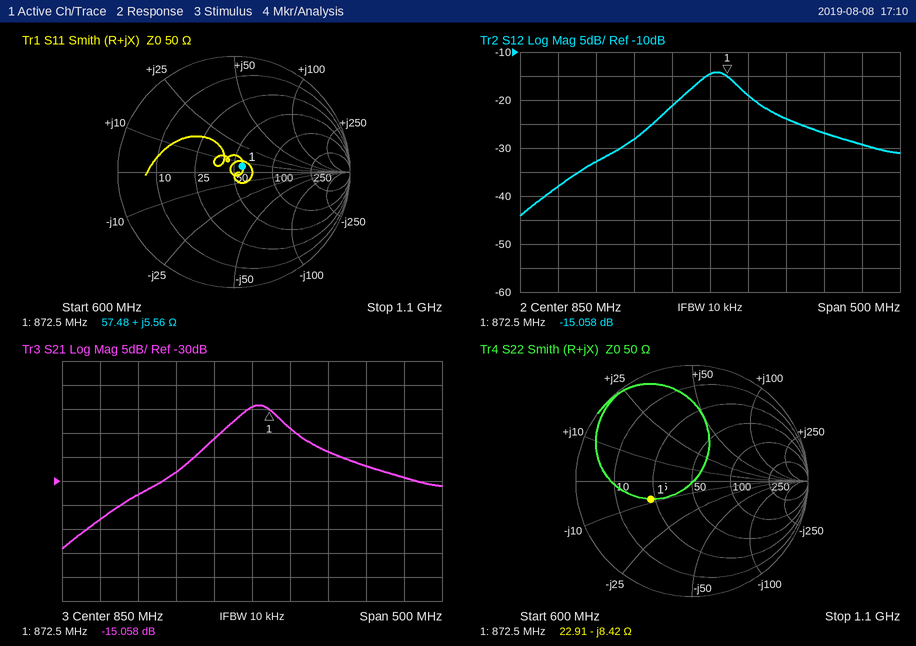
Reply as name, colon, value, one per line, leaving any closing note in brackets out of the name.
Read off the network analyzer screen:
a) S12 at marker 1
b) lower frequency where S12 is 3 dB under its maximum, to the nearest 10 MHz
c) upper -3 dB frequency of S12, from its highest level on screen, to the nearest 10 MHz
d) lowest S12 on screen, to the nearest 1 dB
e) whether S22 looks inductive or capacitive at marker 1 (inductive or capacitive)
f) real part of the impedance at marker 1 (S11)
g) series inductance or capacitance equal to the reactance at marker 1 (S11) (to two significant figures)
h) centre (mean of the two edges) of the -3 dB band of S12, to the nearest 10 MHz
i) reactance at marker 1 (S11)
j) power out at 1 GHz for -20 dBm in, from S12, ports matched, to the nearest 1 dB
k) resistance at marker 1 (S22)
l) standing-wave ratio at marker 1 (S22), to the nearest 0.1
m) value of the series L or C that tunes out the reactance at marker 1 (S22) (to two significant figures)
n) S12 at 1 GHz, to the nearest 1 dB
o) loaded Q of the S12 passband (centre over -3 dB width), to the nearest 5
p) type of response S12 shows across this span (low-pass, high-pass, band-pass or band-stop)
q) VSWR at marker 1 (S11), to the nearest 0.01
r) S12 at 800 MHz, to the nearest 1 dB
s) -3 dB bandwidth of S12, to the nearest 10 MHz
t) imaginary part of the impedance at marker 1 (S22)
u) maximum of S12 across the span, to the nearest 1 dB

S12 at marker 1: -15.058 dB
lower frequency where S12 is 3 dB under its maximum, to the nearest 10 MHz: 830 MHz
upper -3 dB frequency of S12, from its highest level on screen, to the nearest 10 MHz: 890 MHz
lowest S12 on screen, to the nearest 1 dB: -44 dB
whether S22 looks inductive or capacitive at marker 1: capacitive
real part of the impedance at marker 1: 57.48 Ω
series inductance or capacitance equal to the reactance at marker 1 (S11): 1.0 nH
centre (mean of the two edges) of the -3 dB band of S12, to the nearest 10 MHz: 860 MHz
reactance at marker 1: +5.56 Ω
power out at 1 GHz for -20 dBm in, from S12, ports matched, to the nearest 1 dB: -47 dBm
resistance at marker 1: 22.91 Ω
standing-wave ratio at marker 1 (S22), to the nearest 0.1: 2.3
value of the series L or C that tunes out the reactance at marker 1 (S22): 1.5 nH
S12 at 1 GHz, to the nearest 1 dB: -27 dB
loaded Q of the S12 passband (centre over -3 dB width), to the nearest 5: 15
type of response S12 shows across this span: band-pass
VSWR at marker 1 (S11), to the nearest 0.01: 1.19
S12 at 800 MHz, to the nearest 1 dB: -21 dB
-3 dB bandwidth of S12, to the nearest 10 MHz: 60 MHz
imaginary part of the impedance at marker 1: -8.42 Ω
maximum of S12 across the span, to the nearest 1 dB: -14 dB
